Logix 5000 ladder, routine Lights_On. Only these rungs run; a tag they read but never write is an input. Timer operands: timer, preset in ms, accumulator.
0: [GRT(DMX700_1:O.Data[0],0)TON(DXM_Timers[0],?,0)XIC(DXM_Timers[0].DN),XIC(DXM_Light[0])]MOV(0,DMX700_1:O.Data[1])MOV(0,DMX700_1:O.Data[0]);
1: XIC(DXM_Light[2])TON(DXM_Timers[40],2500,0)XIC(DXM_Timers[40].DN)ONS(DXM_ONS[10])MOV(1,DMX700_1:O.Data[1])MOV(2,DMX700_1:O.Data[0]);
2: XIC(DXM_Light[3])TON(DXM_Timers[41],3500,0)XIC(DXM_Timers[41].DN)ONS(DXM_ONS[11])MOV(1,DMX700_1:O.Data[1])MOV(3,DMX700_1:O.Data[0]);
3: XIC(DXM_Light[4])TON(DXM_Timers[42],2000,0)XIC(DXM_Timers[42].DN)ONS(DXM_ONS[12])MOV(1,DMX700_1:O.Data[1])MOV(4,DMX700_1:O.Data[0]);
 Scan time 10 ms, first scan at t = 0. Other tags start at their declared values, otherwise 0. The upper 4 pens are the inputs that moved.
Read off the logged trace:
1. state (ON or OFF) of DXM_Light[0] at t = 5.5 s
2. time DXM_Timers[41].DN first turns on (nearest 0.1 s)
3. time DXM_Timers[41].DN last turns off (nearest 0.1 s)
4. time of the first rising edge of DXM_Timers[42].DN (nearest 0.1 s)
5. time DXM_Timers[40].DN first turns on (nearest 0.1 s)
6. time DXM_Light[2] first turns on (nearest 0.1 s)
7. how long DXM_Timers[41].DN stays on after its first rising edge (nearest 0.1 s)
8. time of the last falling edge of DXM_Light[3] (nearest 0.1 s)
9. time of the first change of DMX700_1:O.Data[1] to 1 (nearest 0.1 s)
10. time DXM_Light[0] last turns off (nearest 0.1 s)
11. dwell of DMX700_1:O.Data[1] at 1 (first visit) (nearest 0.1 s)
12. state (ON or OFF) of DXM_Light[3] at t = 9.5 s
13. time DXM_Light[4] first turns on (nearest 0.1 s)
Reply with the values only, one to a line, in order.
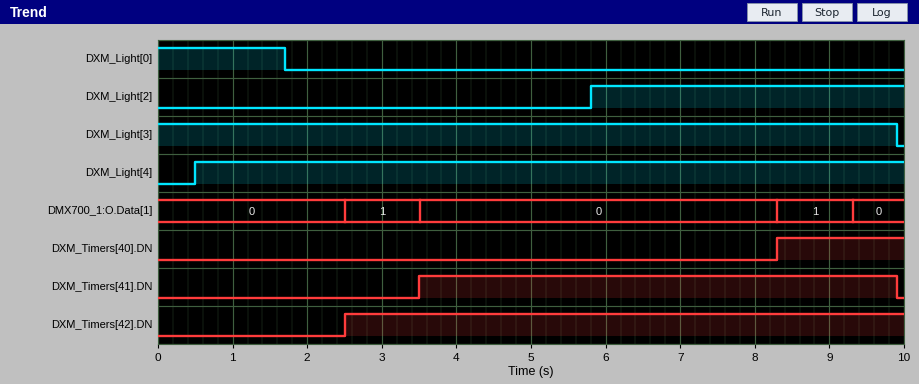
OFF
3.5 s
9.9 s
2.5 s
8.3 s
5.8 s
6.4 s
9.9 s
2.5 s
1.7 s
1.0 s
ON
0.5 s
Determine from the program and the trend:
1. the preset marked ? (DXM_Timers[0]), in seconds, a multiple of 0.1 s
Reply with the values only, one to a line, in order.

1.0 s
